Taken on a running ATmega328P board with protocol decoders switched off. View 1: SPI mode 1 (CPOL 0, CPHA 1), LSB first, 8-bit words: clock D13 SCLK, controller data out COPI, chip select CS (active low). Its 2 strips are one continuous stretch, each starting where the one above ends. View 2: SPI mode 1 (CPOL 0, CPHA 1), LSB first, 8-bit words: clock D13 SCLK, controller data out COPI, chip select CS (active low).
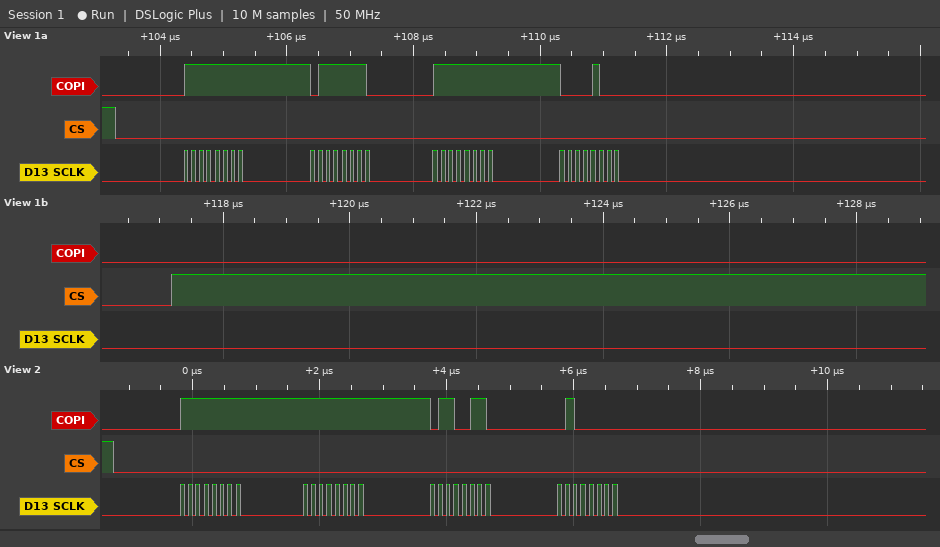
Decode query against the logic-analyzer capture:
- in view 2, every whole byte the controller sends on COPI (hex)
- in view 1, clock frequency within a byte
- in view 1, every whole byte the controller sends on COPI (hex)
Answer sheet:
FF FF 66 02
8 MHz
FF 7E FF 10
